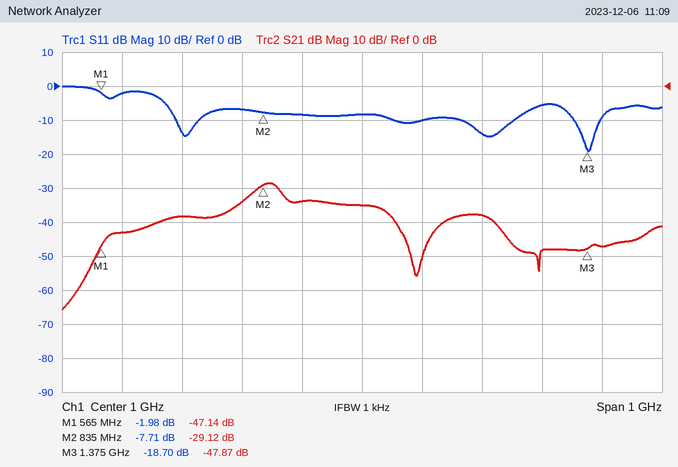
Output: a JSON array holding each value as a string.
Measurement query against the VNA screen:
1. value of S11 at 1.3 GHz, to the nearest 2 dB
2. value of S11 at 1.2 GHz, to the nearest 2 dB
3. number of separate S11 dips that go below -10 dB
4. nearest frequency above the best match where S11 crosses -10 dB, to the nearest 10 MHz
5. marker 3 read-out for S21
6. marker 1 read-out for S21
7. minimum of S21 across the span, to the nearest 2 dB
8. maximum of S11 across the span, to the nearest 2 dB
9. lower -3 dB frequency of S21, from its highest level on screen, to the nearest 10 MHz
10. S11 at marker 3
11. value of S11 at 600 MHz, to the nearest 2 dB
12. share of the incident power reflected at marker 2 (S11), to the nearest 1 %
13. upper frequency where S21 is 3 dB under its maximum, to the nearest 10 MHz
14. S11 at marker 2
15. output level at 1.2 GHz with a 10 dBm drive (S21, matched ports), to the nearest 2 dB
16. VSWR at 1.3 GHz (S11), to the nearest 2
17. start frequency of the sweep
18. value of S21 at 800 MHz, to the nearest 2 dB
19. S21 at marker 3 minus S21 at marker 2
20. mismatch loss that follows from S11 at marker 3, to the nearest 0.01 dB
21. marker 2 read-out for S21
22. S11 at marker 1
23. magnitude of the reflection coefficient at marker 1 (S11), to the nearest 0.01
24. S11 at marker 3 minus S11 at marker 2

["-6 dB", "-14 dB", "3", "1.40 GHz", "-47.87 dB", "-47.14 dB", "-66 dB", "0 dB", "820 MHz", "-18.70 dB", "-2 dB", "17 %", "870 MHz", "-7.71 dB", "-28 dBm", "4", "500 MHz", "-34 dB", "-18.75 dB", "0.06 dB", "-29.12 dB", "-1.98 dB", "0.80", "-10.99 dB"]
